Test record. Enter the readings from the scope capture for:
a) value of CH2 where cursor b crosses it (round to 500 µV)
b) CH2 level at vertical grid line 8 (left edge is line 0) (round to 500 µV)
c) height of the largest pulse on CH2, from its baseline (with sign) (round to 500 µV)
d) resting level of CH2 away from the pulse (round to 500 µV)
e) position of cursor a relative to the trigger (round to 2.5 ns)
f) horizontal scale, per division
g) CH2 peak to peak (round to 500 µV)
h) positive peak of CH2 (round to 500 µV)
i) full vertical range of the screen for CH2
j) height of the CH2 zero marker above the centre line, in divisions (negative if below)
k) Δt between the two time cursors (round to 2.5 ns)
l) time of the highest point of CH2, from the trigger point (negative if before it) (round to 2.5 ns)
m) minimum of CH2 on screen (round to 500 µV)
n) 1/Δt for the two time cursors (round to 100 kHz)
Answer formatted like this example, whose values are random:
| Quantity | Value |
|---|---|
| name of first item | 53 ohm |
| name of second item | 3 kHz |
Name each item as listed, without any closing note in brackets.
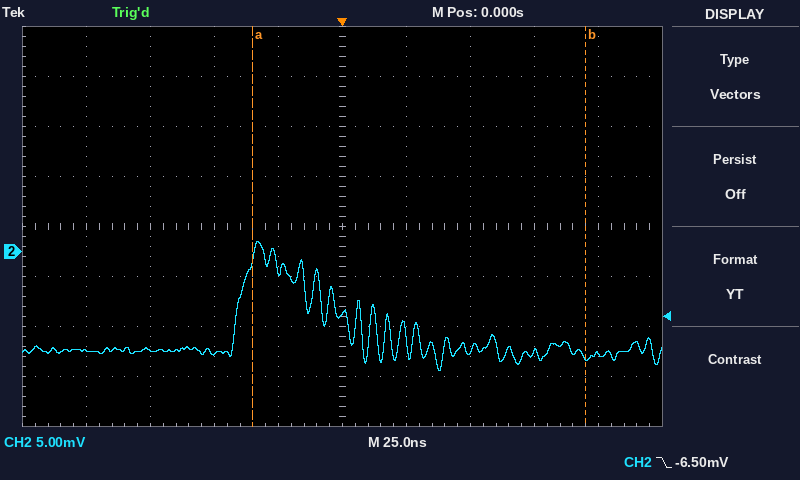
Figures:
| Quantity | Value |
|---|---|
| value of CH2 where cursor b crosses it | -10.5 mV |
| CH2 level at vertical grid line 8 (left edge is line 0) | -10.0 mV |
| height of the largest pulse on CH2, from its baseline (with sign) | +11.0 mV |
| resting level of CH2 away from the pulse | -10.0 mV |
| position of cursor a relative to the trigger | -35.0 ns |
| horizontal scale, per division | 25 ns |
| CH2 peak to peak | 13.0 mV |
| positive peak of CH2 | 1.0 mV |
| full vertical range of the screen for CH2 | 40 mV |
| height of the CH2 zero marker above the centre line, in divisions | -0.5 div |
| Δt between the two time cursors | 130.0 ns |
| time of the highest point of CH2, from the trigger point (negative if before it) | -32.5 ns |
| minimum of CH2 on screen | -12.0 mV |
| 1/Δt for the two time cursors | 7.7 MHz |
